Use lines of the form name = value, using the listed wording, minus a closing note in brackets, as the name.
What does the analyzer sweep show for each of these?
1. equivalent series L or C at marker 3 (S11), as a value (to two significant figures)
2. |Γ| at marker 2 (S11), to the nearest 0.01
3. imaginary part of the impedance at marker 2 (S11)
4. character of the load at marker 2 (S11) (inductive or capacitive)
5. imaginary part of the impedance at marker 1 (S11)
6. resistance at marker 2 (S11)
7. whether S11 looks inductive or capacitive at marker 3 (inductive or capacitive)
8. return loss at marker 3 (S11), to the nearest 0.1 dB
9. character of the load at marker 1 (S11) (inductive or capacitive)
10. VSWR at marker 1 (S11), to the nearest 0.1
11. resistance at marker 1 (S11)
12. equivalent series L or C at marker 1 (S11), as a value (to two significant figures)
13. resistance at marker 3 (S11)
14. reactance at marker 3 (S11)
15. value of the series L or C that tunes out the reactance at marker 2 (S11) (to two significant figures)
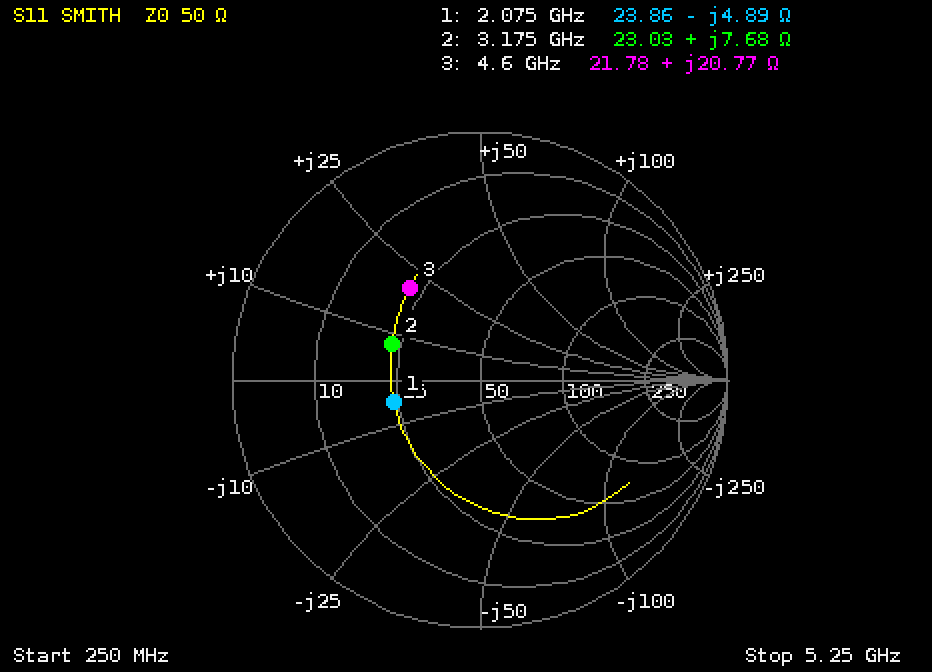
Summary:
equivalent series L or C at marker 3 (S11), as a value = 720 pH
|Γ| at marker 2 (S11), to the nearest 0.01 = 0.38
imaginary part of the impedance at marker 2 = +7.68 Ω
character of the load at marker 2 (S11) = inductive
imaginary part of the impedance at marker 1 = -4.89 Ω
resistance at marker 2 = 23.03 Ω
whether S11 looks inductive or capacitive at marker 3 = inductive
return loss at marker 3 (S11), to the nearest 0.1 dB = 6.6 dB
character of the load at marker 1 (S11) = capacitive
VSWR at marker 1 (S11), to the nearest 0.1 = 2.1
resistance at marker 1 = 23.86 Ω
equivalent series L or C at marker 1 (S11), as a value = 16 pF
resistance at marker 3 = 21.78 Ω
reactance at marker 3 = +20.77 Ω
value of the series L or C that tunes out the reactance at marker 2 (S11) = 6.5 pF
